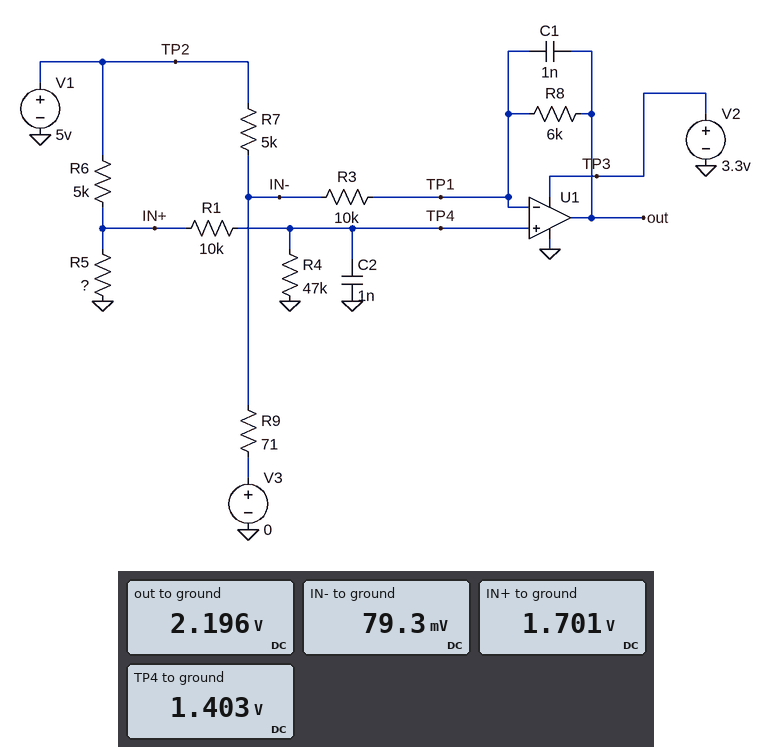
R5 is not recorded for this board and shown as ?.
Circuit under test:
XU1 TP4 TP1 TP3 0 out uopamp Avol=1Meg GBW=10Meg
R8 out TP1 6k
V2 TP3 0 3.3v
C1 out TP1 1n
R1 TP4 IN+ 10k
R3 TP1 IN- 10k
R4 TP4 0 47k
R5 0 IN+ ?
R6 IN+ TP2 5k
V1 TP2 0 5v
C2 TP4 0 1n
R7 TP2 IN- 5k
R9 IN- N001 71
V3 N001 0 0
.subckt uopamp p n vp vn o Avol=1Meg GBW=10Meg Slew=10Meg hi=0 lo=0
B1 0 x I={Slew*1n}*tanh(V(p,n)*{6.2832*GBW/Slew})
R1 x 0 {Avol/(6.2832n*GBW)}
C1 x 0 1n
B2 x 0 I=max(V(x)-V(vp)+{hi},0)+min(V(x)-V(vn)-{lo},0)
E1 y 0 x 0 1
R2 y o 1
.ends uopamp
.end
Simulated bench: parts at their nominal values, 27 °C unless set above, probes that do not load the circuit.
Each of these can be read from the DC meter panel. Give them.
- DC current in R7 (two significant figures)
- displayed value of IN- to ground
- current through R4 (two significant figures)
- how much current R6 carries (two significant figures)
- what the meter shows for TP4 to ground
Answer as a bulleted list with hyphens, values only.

- 980 µA
- 79.3 mV
- 30 µA
- 660 µA
- 1.403 V
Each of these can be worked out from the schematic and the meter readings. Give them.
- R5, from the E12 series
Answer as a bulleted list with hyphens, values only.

- 2.7 kΩ
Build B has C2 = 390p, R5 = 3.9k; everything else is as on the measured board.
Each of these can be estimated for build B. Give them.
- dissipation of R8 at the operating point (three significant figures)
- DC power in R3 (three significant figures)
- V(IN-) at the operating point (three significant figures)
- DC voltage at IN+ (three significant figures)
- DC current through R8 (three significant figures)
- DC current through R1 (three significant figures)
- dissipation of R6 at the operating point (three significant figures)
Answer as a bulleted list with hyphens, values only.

- 165 µW
- 275 µW
- 81.6 mV
- 2.11 V
- 166 µA
- 37.0 µA
- 1.67 mW
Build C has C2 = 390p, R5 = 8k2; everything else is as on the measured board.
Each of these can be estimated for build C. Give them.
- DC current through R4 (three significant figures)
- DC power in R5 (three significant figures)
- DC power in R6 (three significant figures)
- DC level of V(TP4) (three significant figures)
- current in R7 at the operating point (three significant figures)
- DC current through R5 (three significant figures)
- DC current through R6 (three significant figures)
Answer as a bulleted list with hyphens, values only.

- 51.7 µA
- 1.06 mW
- 844 µW
- 2.43 V
- 983 µA
- 359 µA
- 411 µA
